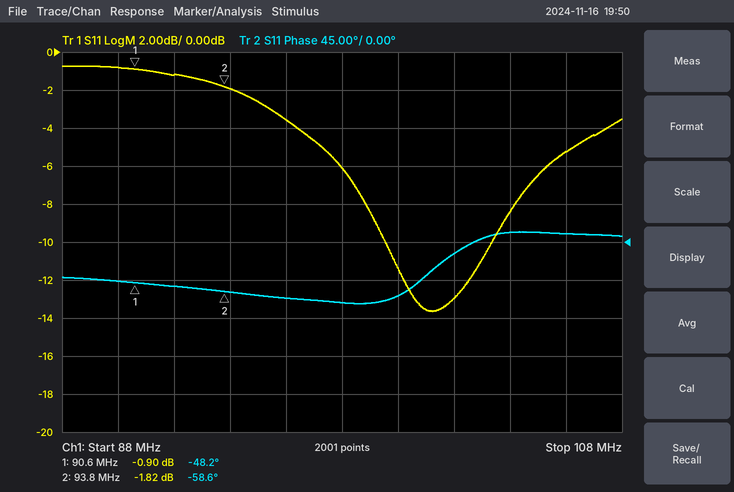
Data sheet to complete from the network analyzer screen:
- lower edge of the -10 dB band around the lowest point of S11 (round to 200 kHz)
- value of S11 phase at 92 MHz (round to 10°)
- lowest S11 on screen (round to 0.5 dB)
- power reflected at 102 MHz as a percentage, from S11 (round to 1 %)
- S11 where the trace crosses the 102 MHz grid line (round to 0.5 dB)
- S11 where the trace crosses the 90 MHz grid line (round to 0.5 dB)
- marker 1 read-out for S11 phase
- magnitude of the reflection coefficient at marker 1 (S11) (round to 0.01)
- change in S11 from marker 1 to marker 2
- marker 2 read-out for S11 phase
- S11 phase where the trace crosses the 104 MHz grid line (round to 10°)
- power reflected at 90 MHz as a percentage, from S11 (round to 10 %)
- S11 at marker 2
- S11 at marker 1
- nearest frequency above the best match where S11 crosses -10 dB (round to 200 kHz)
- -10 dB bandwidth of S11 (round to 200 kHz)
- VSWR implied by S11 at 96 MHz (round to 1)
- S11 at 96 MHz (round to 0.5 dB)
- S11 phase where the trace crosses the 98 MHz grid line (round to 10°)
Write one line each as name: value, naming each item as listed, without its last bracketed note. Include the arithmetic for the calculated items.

lower edge of the -10 dB band around the lowest point of S11: 99.6 MHz
value of S11 phase at 92 MHz: -50°
lowest S11 on screen: -13.5 dB
power reflected at 102 MHz as a percentage, from S11: 10^(-13/10) ≈ 5 %
S11 where the trace crosses the 102 MHz grid line: -13.0 dB
S11 where the trace crosses the 90 MHz grid line: -1.0 dB
marker 1 read-out for S11 phase: -48.2°
magnitude of the reflection coefficient at marker 1 (S11): 10^(-0.9/20) ≈ 0.90
change in S11 from marker 1 to marker 2: -1.82 − (-0.9) = -0.92 dB
marker 2 read-out for S11 phase: -58.6°
S11 phase where the trace crosses the 104 MHz grid line: 10°
power reflected at 90 MHz as a percentage, from S11: 10^(-1/10) ≈ 79.4 %, so 80 % to the nearest 10 %
S11 at marker 2: -1.82 dB
S11 at marker 1: -0.90 dB
nearest frequency above the best match where S11 crosses -10 dB: 103.4 MHz
-10 dB bandwidth of S11: 103.4 MHz − 99.6 MHz = 3.8 MHz
VSWR implied by S11 at 96 MHz: |Γ| = 10^(-3.5/20) = 0.6683; VSWR = (1 + 0.6683)/(1 − 0.6683) ≈ 5
S11 at 96 MHz: -3.5 dB
S11 phase where the trace crosses the 98 MHz grid line: -70°
